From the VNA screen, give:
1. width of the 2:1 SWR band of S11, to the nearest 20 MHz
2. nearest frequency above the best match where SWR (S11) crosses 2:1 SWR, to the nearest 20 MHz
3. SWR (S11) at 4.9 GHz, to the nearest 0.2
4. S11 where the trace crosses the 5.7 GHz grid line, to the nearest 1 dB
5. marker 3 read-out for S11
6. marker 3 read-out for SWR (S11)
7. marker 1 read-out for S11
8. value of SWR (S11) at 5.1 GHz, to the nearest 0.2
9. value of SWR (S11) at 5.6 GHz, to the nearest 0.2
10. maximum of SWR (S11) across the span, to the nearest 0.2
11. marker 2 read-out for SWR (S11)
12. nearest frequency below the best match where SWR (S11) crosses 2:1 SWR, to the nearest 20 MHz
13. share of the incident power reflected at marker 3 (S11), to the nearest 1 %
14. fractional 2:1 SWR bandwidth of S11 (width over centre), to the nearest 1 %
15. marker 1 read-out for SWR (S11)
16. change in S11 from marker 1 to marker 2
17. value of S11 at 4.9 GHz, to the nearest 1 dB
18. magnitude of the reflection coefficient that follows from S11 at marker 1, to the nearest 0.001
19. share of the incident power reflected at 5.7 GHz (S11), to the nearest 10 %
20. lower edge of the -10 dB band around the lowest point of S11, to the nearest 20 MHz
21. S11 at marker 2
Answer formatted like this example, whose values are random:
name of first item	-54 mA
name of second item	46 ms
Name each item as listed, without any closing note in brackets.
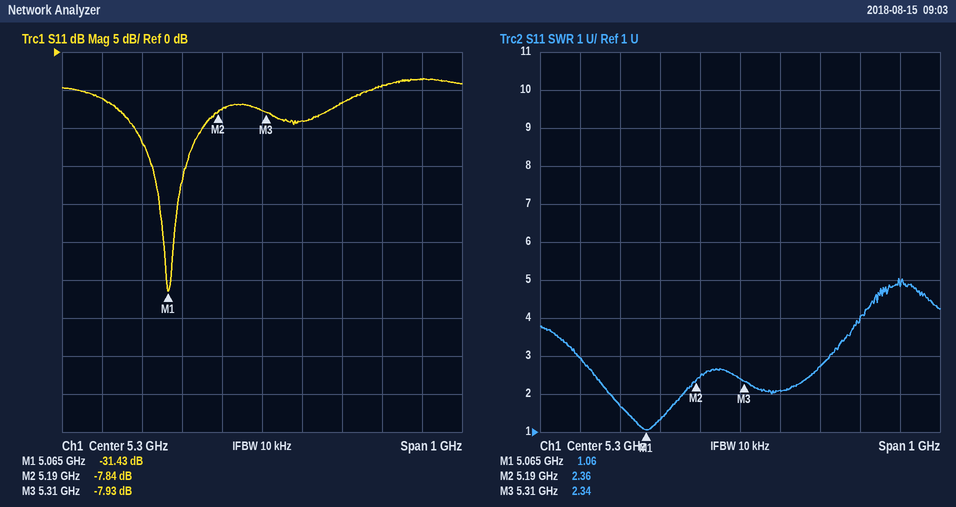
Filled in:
width of the 2:1 SWR band of S11, to the nearest 20 MHz	180 MHz
nearest frequency above the best match where SWR (S11) crosses 2:1 SWR, to the nearest 20 MHz	5.16 GHz
SWR (S11) at 4.9 GHz, to the nearest 0.2	3.0
S11 where the trace crosses the 5.7 GHz grid line, to the nearest 1 dB	-4 dB
marker 3 read-out for S11	-7.93 dB
marker 3 read-out for SWR	2.34
marker 1 read-out for S11	-31.43 dB
value of SWR (S11) at 5.1 GHz, to the nearest 0.2	1.4
value of SWR (S11) at 5.6 GHz, to the nearest 0.2	4.0
maximum of SWR (S11) across the span, to the nearest 0.2	5.0
marker 2 read-out for SWR	2.36
nearest frequency below the best match where SWR (S11) crosses 2:1 SWR, to the nearest 20 MHz	4.98 GHz
share of the incident power reflected at marker 3 (S11), to the nearest 1 %	16 %
fractional 2:1 SWR bandwidth of S11 (width over centre), to the nearest 1 %	4 %
marker 1 read-out for SWR	1.06
change in S11 from marker 1 to marker 2	23.59 dB
value of S11 at 4.9 GHz, to the nearest 1 dB	-6 dB
magnitude of the reflection coefficient that follows from S11 at marker 1, to the nearest 0.001	0.027
share of the incident power reflected at 5.7 GHz (S11), to the nearest 10 %	40 %
lower edge of the -10 dB band around the lowest point of S11, to the nearest 20 MHz	4.98 GHz
S11 at marker 2	-7.84 dB
